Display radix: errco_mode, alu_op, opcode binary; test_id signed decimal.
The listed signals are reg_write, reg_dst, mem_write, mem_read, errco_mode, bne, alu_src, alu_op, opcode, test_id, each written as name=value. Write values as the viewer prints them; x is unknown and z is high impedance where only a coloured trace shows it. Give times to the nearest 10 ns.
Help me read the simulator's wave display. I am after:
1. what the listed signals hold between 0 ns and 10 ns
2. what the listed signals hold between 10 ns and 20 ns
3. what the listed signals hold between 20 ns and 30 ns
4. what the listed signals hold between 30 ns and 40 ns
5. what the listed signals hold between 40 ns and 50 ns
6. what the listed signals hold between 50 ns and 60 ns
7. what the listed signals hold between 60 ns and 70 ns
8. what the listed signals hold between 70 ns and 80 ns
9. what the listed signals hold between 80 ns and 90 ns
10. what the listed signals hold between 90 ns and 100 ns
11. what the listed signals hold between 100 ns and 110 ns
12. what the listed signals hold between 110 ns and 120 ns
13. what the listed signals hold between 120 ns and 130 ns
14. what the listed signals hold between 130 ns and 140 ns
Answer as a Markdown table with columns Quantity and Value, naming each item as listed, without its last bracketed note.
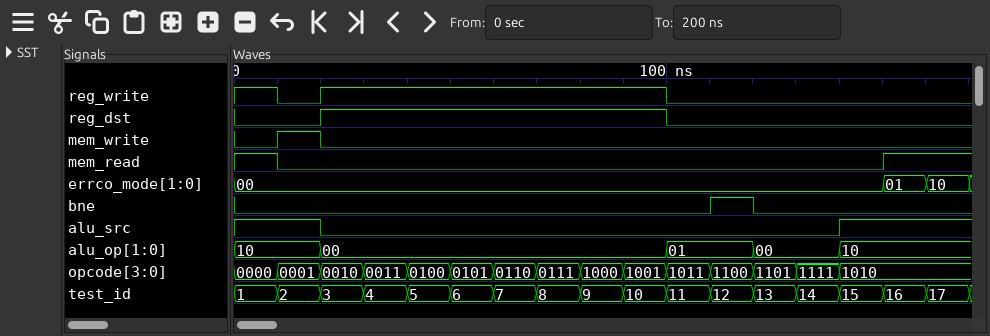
| Quantity | Value |
|---|---|
| what the listed signals hold between 0 ns and 10 ns | reg_write=1, reg_dst=0, mem_write=0, mem_read=1, errco_mode=00, bne=0, alu_src=1, alu_op=10, opcode=0000, test_id=1 |
| what the listed signals hold between 10 ns and 20 ns | reg_write=0, reg_dst=0, mem_write=1, mem_read=0, errco_mode=00, bne=0, alu_src=1, alu_op=10, opcode=0001, test_id=2 |
| what the listed signals hold between 20 ns and 30 ns | reg_write=1, reg_dst=1, mem_write=0, mem_read=0, errco_mode=00, bne=0, alu_src=0, alu_op=00, opcode=0010, test_id=3 |
| what the listed signals hold between 30 ns and 40 ns | reg_write=1, reg_dst=1, mem_write=0, mem_read=0, errco_mode=00, bne=0, alu_src=0, alu_op=00, opcode=0011, test_id=4 |
| what the listed signals hold between 40 ns and 50 ns | reg_write=1, reg_dst=1, mem_write=0, mem_read=0, errco_mode=00, bne=0, alu_src=0, alu_op=00, opcode=0100, test_id=5 |
| what the listed signals hold between 50 ns and 60 ns | reg_write=1, reg_dst=1, mem_write=0, mem_read=0, errco_mode=00, bne=0, alu_src=0, alu_op=00, opcode=0101, test_id=6 |
| what the listed signals hold between 60 ns and 70 ns | reg_write=1, reg_dst=1, mem_write=0, mem_read=0, errco_mode=00, bne=0, alu_src=0, alu_op=00, opcode=0110, test_id=7 |
| what the listed signals hold between 70 ns and 80 ns | reg_write=1, reg_dst=1, mem_write=0, mem_read=0, errco_mode=00, bne=0, alu_src=0, alu_op=00, opcode=0111, test_id=8 |
| what the listed signals hold between 80 ns and 90 ns | reg_write=1, reg_dst=1, mem_write=0, mem_read=0, errco_mode=00, bne=0, alu_src=0, alu_op=00, opcode=1000, test_id=9 |
| what the listed signals hold between 90 ns and 100 ns | reg_write=1, reg_dst=1, mem_write=0, mem_read=0, errco_mode=00, bne=0, alu_src=0, alu_op=00, opcode=1001, test_id=10 |
| what the listed signals hold between 100 ns and 110 ns | reg_write=0, reg_dst=0, mem_write=0, mem_read=0, errco_mode=00, bne=0, alu_src=0, alu_op=01, opcode=1011, test_id=11 |
| what the listed signals hold between 110 ns and 120 ns | reg_write=0, reg_dst=0, mem_write=0, mem_read=0, errco_mode=00, bne=1, alu_src=0, alu_op=01, opcode=1100, test_id=12 |
| what the listed signals hold between 120 ns and 130 ns | reg_write=0, reg_dst=0, mem_write=0, mem_read=0, errco_mode=00, bne=0, alu_src=0, alu_op=00, opcode=1101, test_id=13 |
| what the listed signals hold between 130 ns and 140 ns | reg_write=0, reg_dst=0, mem_write=0, mem_read=0, errco_mode=00, bne=0, alu_src=0, alu_op=00, opcode=1111, test_id=14 |
